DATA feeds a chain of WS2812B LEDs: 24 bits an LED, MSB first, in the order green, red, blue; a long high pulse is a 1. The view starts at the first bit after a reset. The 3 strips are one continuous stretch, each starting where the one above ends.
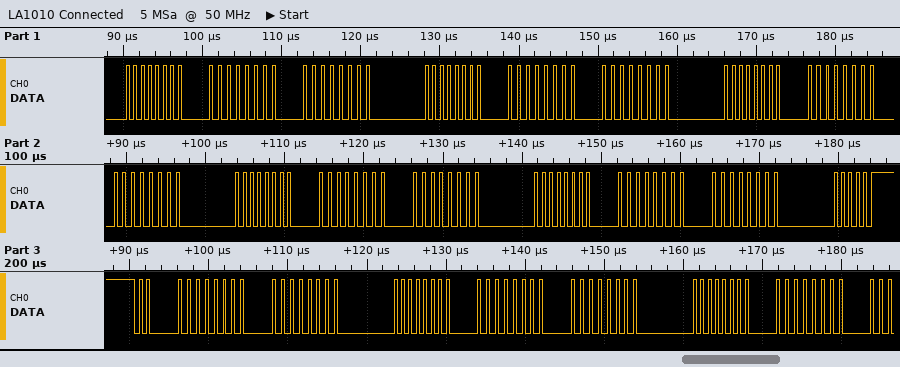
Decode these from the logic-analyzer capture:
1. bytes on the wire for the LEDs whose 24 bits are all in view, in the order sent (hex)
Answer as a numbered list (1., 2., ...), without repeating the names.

1. 00 00 00 00 00 00 00 00 00 00 00 00 00 00 00 04 00 00 00 00 00
